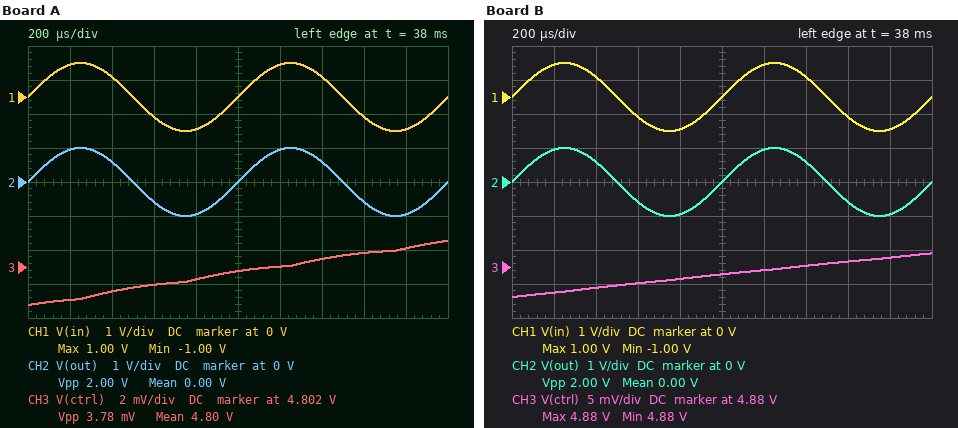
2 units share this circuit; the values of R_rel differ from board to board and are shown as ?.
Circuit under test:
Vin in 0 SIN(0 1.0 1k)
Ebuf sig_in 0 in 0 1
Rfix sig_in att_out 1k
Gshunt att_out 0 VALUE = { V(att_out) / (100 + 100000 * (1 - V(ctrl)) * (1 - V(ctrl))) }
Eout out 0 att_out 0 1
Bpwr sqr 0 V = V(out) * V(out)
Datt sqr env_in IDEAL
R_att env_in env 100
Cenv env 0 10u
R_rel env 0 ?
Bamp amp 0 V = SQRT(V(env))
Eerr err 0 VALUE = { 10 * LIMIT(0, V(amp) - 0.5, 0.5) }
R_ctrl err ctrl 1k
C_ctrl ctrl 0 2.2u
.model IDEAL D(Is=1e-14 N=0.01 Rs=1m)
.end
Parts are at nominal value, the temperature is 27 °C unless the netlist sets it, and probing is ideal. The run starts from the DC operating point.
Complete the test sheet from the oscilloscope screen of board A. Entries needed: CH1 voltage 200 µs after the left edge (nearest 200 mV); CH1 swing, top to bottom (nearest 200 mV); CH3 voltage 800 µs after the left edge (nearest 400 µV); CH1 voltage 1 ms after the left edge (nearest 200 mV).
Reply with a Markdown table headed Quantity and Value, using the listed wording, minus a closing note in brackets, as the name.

| Quantity | Value |
|---|---|
| CH1 voltage 200 µs after the left edge | 1.0 V |
| CH1 swing, top to bottom | 2.0 V |
| CH3 voltage 800 µs after the left edge | 4.8012 V |
| CH1 voltage 1 ms after the left edge | 0 V |
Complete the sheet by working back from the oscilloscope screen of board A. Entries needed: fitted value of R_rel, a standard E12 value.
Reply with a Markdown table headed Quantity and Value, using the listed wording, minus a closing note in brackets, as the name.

| Quantity | Value |
|---|---|
| fitted value of R_rel, a standard E12 value | 47 kΩ |
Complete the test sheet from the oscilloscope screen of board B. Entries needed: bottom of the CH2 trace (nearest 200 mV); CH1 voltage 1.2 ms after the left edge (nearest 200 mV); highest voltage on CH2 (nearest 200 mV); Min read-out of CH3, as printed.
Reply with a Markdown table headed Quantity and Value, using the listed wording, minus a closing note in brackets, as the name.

| Quantity | Value |
|---|---|
| bottom of the CH2 trace | -1.0 V |
| CH1 voltage 1.2 ms after the left edge | 1.0 V |
| highest voltage on CH2 | 1.0 V |
| Min read-out of CH3, as printed | 4.88 V |
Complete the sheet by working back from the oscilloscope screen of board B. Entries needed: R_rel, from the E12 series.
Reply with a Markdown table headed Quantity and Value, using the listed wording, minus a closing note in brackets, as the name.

| Quantity | Value |
|---|---|
| R_rel, from the E12 series | 330 kΩ |
